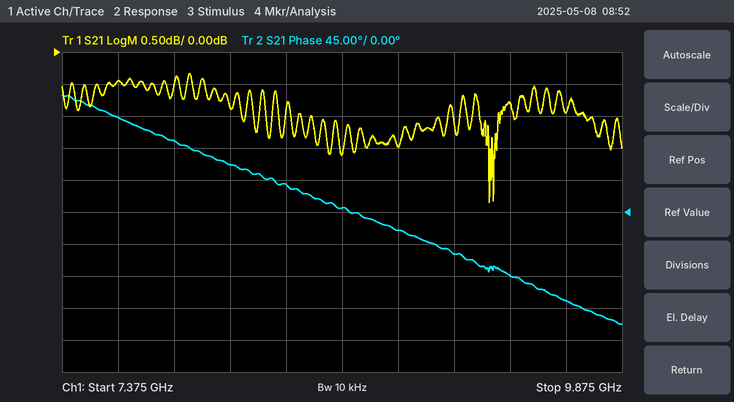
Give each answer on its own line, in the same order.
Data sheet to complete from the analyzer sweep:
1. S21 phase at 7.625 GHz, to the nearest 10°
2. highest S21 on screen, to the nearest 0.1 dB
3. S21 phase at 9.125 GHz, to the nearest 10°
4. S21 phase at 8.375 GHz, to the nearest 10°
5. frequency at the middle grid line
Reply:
130°
-0.3 dB
-60°
40°
8.625 GHz
